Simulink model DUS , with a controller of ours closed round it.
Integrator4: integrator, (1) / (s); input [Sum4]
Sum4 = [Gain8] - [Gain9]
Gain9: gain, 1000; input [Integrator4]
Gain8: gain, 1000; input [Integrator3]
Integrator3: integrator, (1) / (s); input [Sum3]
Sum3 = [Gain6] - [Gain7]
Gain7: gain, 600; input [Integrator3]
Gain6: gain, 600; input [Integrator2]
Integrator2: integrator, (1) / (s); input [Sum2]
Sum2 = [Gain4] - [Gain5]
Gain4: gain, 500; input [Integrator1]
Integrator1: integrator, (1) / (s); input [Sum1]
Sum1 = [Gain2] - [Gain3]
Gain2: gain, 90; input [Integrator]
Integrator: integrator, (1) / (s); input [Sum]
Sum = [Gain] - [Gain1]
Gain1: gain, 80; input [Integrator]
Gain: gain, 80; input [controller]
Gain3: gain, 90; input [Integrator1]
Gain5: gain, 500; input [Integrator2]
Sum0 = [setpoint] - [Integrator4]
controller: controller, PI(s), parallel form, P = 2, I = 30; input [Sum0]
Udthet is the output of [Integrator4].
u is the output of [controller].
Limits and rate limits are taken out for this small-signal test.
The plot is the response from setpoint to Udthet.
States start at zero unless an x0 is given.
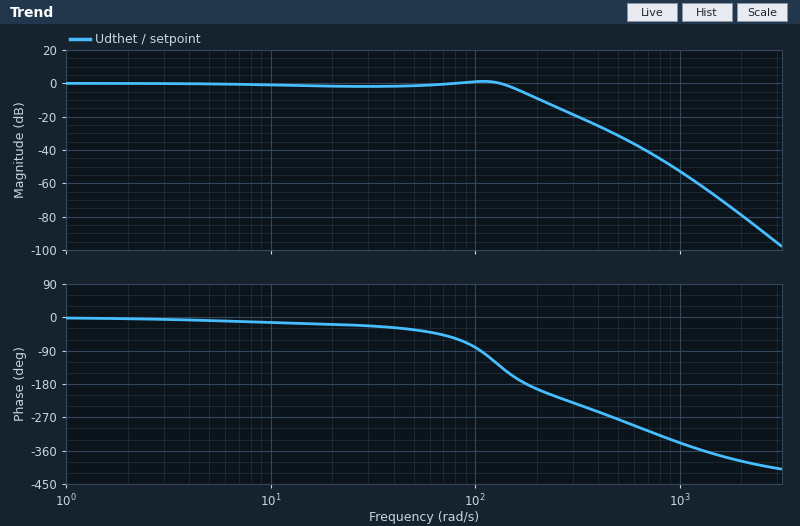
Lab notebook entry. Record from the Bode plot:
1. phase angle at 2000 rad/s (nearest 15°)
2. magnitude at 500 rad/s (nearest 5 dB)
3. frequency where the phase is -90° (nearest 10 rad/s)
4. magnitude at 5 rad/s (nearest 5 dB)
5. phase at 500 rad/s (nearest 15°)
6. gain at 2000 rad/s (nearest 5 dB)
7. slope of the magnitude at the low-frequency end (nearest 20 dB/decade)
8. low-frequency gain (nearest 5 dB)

-390°
-30 dB
110 rad/s
0 dB
-270°
-80 dB
0 dB/decade
0 dB
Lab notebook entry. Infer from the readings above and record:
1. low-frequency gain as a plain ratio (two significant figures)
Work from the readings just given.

1.0
